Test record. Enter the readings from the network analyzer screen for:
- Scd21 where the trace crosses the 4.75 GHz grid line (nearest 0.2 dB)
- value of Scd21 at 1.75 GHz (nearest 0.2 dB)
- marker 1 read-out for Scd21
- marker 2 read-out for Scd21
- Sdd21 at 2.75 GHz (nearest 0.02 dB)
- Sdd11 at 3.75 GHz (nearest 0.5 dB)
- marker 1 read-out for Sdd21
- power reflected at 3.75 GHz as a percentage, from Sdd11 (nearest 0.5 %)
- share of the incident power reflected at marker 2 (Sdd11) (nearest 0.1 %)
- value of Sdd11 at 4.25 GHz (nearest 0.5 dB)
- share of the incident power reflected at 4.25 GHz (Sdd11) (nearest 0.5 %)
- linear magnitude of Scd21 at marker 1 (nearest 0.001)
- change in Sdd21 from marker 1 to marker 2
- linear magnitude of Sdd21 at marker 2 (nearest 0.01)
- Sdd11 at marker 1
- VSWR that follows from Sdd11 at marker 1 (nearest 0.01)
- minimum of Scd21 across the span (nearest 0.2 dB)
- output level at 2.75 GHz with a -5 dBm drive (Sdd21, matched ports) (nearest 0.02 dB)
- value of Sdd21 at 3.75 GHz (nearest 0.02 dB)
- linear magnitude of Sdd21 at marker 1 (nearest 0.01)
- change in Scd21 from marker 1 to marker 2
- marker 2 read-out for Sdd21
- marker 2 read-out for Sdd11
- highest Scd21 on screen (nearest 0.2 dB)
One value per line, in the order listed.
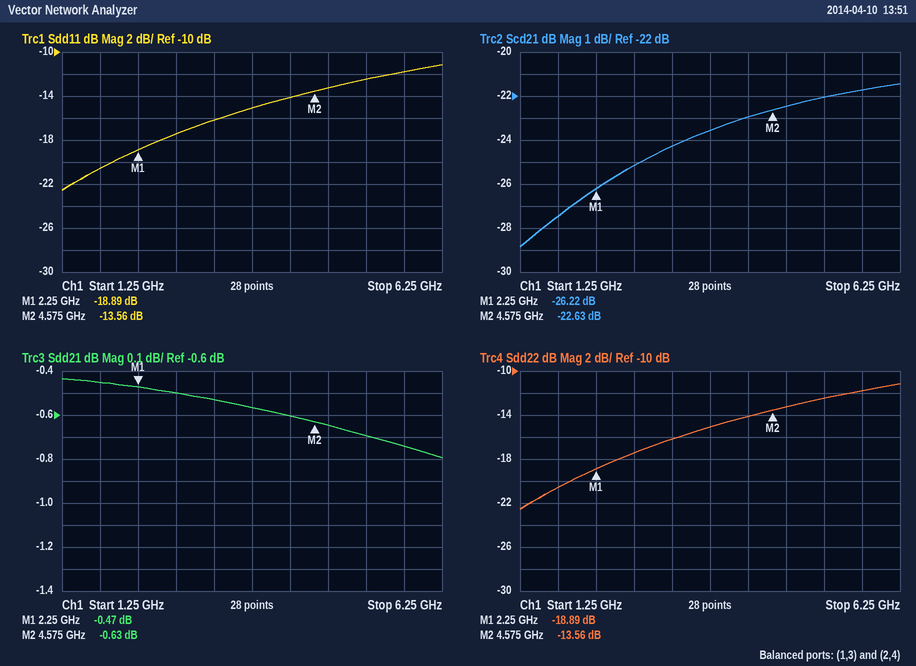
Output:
-22.4 dB
-27.4 dB
-26.22 dB
-22.63 dB
-0.50 dB
-15.0 dB
-0.47 dB
3.0 %
4.4 %
-14.0 dB
4.0 %
0.049
-0.16 dB
0.93
-18.89 dB
1.26
-28.8 dB
-5.50 dBm
-0.56 dB
0.95
3.59 dB
-0.63 dB
-13.56 dB
-21.4 dB
